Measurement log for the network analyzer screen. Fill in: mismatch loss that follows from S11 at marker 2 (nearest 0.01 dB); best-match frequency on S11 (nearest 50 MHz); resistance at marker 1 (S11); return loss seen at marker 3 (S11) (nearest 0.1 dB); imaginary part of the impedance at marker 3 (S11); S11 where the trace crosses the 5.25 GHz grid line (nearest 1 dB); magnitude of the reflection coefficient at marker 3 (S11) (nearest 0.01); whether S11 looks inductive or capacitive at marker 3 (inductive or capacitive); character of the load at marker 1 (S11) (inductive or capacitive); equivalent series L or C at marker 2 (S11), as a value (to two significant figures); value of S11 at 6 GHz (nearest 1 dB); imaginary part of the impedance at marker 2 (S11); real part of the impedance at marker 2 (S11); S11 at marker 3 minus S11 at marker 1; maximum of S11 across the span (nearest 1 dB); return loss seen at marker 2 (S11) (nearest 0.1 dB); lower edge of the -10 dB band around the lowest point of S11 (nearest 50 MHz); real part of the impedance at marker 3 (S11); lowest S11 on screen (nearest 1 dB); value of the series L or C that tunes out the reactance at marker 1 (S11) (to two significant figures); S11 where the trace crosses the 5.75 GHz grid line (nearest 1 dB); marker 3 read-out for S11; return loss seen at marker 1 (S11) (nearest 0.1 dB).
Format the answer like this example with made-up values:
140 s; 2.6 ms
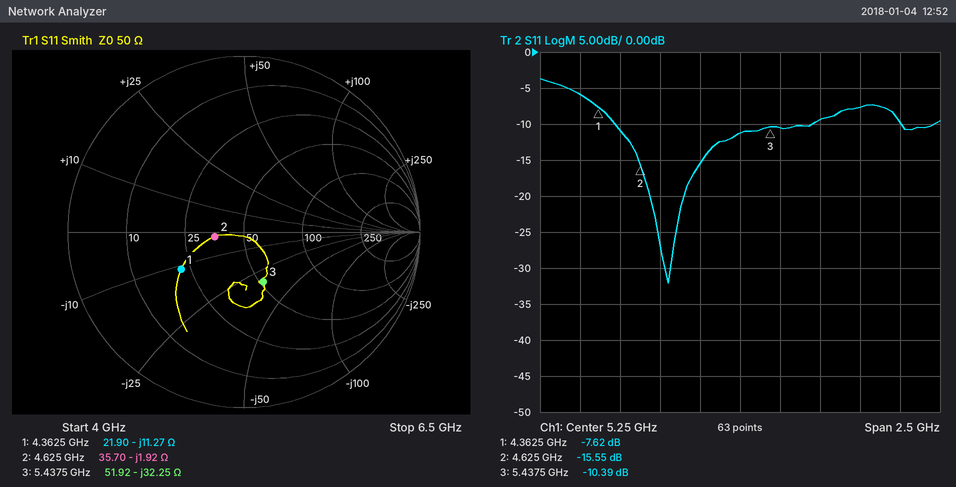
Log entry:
0.12 dB; 4.80 GHz; 21.90 Ω; 10.4 dB; -32.25 Ω; -11 dB; 0.30; capacitive; capacitive; 18 pF; -8 dB; -1.92 Ω; 35.70 Ω; -2.77 dB; -4 dB; 15.5 dB; 4.45 GHz; 51.92 Ω; -32 dB; 410 pH; -9 dB; -10.39 dB; 7.6 dB
